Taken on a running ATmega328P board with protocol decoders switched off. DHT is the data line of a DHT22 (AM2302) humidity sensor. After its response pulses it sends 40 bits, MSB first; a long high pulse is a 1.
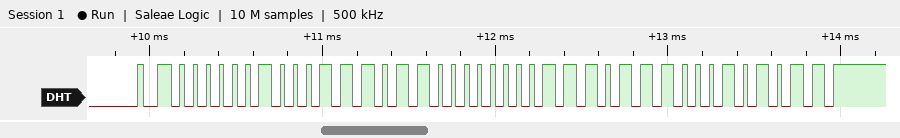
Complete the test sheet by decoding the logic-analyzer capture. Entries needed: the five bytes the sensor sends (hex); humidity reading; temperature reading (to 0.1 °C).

02 3B 00 EE 2B
57.1 %
23.8 °C
